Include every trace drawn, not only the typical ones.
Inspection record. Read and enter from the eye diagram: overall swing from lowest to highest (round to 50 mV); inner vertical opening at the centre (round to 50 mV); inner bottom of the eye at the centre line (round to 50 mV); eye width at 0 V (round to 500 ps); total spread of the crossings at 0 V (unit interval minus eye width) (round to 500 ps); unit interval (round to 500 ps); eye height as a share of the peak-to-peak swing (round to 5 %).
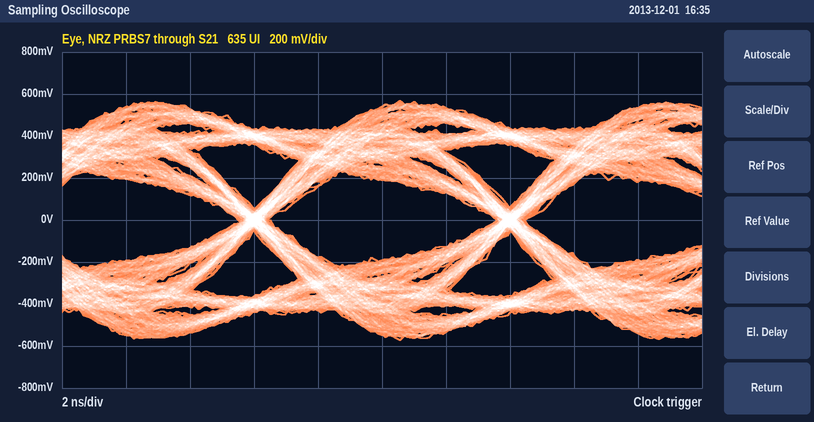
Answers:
1.15 V
400 mV
-200 mV
7.0 ns
1.0 ns
8.0 ns
35 %
